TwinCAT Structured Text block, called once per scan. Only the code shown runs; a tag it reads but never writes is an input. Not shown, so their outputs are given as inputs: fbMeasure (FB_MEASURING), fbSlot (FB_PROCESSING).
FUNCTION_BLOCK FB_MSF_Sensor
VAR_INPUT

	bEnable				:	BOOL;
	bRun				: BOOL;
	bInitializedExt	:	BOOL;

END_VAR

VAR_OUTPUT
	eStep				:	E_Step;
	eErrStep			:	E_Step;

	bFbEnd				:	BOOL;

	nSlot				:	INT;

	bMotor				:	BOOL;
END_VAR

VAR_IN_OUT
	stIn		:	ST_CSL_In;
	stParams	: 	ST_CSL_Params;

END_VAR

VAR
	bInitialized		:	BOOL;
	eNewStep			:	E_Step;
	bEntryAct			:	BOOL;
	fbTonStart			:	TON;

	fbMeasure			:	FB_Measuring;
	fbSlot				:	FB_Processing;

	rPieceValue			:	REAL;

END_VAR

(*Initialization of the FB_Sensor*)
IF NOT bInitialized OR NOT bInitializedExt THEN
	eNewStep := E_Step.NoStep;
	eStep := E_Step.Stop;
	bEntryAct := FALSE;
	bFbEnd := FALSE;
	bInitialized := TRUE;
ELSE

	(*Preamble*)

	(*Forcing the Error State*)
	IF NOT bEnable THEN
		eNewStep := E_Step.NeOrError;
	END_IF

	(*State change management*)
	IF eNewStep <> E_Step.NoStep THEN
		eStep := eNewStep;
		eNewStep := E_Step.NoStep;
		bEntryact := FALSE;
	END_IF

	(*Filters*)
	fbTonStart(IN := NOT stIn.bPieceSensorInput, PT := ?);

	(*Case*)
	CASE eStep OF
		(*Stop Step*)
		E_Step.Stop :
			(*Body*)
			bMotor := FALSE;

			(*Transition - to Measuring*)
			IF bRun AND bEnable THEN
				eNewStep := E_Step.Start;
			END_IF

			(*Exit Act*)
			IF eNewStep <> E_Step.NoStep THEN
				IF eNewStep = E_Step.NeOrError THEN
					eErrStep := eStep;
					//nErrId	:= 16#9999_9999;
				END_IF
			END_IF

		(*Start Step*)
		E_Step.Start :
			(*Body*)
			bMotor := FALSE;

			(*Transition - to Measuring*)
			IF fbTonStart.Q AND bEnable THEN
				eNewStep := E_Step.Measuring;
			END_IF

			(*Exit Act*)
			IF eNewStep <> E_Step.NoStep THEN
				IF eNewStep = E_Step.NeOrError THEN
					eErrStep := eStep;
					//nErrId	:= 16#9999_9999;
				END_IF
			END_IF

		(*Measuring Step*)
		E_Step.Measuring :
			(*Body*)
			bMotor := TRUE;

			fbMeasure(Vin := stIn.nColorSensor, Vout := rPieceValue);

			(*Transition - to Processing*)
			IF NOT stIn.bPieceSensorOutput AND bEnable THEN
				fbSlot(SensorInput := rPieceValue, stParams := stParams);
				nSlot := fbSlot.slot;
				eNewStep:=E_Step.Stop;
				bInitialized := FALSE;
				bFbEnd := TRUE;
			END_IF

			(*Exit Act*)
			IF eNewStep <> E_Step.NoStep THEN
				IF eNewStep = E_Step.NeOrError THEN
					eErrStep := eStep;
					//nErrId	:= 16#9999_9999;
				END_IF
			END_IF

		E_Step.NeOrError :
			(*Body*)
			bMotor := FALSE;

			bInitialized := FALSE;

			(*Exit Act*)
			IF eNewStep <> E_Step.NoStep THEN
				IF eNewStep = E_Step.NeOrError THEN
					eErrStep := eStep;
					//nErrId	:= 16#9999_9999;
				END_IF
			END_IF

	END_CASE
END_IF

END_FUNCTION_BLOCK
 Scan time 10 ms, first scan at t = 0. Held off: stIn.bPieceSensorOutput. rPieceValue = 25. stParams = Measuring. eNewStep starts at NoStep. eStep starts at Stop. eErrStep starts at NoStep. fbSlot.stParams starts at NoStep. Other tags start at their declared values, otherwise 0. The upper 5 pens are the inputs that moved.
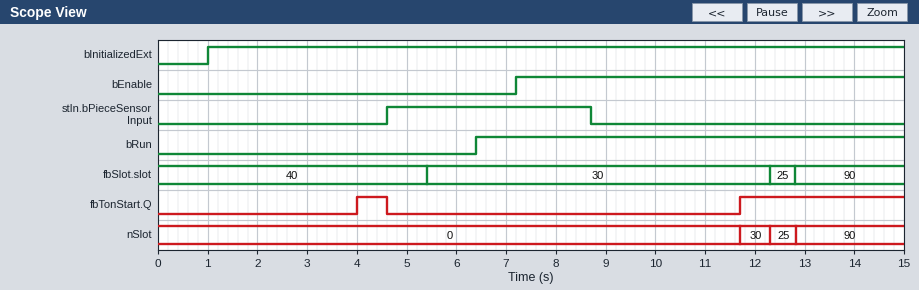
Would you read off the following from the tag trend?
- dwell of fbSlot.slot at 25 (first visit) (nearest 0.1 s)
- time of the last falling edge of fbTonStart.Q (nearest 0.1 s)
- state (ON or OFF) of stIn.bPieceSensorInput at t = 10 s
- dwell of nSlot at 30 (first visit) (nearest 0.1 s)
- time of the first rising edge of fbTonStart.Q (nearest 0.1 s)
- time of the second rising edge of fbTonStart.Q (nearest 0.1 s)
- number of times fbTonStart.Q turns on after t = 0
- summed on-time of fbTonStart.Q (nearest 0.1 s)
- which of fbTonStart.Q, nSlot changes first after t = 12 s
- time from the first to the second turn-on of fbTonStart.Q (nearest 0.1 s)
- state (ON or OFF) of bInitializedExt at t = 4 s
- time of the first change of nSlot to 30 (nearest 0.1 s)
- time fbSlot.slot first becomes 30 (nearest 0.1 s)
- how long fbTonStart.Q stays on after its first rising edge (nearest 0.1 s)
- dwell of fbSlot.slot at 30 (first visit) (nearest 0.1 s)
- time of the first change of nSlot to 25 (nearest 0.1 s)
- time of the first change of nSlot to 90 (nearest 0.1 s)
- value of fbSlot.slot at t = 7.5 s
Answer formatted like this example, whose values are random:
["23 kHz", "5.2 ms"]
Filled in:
["0.5 s", "4.6 s", "OFF", "0.6 s", "4.0 s", "11.7 s", "2", "3.9 s", "nSlot", "7.7 s", "ON", "11.7 s", "5.4 s", "0.6 s", "6.9 s", "12.3 s", "12.8 s", "30"]
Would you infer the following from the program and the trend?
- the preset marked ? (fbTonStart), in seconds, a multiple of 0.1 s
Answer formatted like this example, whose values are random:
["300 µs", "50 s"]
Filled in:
["3.0 s"]
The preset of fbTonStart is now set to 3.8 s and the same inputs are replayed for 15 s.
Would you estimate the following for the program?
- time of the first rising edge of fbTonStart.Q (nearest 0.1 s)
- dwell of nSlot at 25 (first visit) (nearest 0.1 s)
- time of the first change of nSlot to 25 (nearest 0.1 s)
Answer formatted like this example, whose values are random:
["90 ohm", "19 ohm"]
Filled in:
["12.5 s", "0.3 s", "12.5 s"]
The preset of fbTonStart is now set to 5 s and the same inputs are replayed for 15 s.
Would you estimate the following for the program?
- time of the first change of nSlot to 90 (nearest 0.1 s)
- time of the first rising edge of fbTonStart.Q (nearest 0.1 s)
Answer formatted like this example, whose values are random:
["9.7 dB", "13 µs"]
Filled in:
["13.7 s", "13.7 s"]
